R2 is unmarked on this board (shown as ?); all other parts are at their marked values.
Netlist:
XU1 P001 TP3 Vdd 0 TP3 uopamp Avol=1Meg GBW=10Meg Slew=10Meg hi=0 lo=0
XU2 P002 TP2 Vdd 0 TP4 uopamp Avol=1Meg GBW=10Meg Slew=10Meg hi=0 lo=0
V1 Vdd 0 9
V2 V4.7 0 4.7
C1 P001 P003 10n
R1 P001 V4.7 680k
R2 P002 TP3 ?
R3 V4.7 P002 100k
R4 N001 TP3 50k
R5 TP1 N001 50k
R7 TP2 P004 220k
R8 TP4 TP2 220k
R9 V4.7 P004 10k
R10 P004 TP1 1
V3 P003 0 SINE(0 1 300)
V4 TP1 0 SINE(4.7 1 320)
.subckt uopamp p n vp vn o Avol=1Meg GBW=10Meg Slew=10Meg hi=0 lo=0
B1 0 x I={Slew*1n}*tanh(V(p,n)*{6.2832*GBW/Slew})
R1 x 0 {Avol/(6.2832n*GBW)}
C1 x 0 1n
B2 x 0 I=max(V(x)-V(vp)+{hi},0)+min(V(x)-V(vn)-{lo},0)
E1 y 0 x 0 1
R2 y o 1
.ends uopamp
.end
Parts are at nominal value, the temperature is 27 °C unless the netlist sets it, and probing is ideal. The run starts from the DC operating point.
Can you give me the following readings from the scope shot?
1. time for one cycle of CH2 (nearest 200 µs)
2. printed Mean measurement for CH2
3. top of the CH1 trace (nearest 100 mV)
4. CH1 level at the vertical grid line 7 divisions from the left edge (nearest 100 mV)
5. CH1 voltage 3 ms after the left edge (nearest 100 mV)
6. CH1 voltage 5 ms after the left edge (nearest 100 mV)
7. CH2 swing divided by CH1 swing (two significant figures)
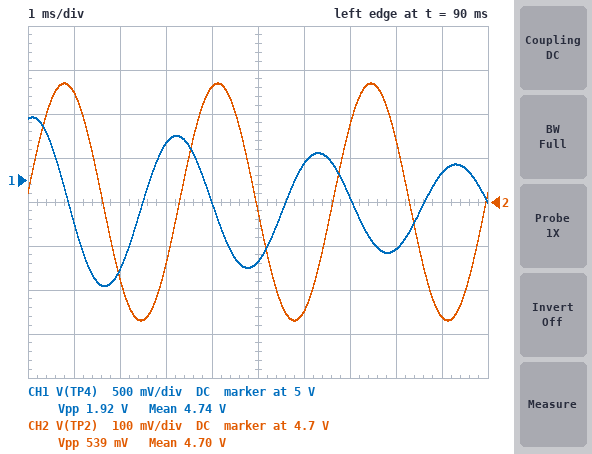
3.4 ms
4.70 V
5.7 V
4.8 V
5.4 V
4.1 V
0.28
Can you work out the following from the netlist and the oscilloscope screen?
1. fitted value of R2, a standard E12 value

270 kΩ
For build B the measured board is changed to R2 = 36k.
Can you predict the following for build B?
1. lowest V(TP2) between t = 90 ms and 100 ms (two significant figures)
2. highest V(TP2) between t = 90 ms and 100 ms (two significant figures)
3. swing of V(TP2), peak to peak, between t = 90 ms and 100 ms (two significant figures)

4.0 V
5.4 V
1.5 V
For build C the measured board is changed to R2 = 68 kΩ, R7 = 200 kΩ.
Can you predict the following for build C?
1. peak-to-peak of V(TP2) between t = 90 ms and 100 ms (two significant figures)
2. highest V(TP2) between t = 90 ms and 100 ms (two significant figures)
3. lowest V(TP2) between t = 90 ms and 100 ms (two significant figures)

1.2 V
5.3 V
4.1 V
